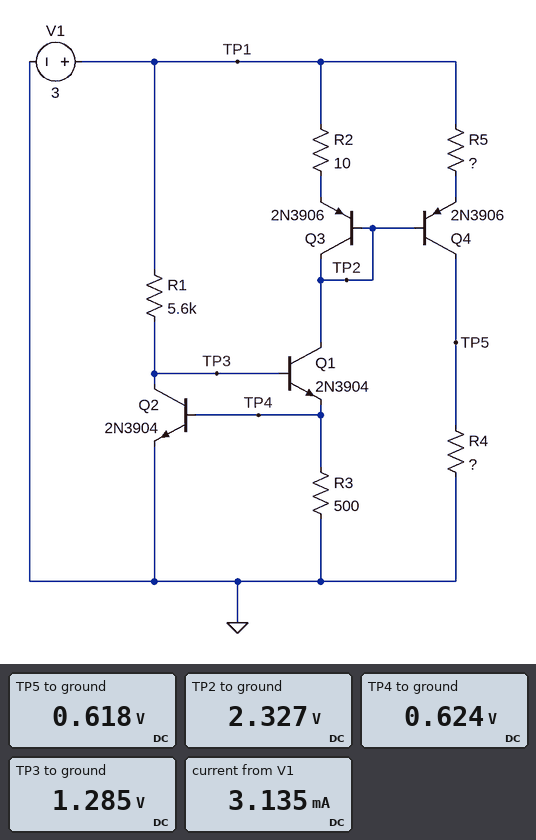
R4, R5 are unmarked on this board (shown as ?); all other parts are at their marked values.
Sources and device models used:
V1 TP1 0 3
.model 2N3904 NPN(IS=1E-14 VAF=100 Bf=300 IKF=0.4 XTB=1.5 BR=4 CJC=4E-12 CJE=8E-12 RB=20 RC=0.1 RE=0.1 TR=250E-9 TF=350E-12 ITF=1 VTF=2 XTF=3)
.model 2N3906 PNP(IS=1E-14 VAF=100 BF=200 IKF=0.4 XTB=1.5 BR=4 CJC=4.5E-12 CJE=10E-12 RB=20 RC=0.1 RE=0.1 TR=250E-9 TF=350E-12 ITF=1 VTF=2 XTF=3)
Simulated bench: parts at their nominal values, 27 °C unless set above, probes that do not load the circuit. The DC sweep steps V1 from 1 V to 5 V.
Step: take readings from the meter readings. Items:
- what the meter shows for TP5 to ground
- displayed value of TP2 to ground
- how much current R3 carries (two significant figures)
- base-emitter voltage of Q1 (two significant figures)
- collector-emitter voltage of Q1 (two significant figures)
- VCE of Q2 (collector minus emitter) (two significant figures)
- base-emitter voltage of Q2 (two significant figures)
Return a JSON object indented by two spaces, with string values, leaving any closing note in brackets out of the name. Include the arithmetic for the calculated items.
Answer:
{
  "what the meter shows for TP5 to ground": "0.618 V",
  "displayed value of TP2 to ground": "2.327 V",
  "how much current R3 carries": "(624 mV) / 500 Ω = 1.2 mA",
  "base-emitter voltage of Q1": "1.285 V - 624 mV = 660 mV",
  "collector-emitter voltage of Q1": "2.327 V - 624 mV = 1.7 V",
  "VCE of Q2 (collector minus emitter)": "1.285 V = 1.3 V",
  "base-emitter voltage of Q2": "624 mV = 620 mV"
}
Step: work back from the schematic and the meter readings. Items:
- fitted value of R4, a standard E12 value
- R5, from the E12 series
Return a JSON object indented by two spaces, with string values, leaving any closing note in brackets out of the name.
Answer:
{
  "fitted value of R4, a standard E12 value": "390 Ω",
  "R5, from the E12 series": "3.9 Ω"
}
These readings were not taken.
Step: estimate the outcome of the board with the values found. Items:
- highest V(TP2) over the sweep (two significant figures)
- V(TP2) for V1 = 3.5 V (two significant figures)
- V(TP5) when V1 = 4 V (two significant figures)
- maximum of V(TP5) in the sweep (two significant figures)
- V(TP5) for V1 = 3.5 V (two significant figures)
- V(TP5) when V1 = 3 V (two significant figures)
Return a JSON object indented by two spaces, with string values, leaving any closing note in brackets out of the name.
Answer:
{
  "highest V(TP2) over the sweep": "4.3 V",
  "V(TP2) for V1 = 3.5 V": "2.8 V",
  "V(TP5) when V1 = 4 V": "640 mV",
  "maximum of V(TP5) in the sweep": "650 mV",
  "V(TP5) for V1 = 3.5 V": "630 mV",
  "V(TP5) when V1 = 3 V": "620 mV"
}
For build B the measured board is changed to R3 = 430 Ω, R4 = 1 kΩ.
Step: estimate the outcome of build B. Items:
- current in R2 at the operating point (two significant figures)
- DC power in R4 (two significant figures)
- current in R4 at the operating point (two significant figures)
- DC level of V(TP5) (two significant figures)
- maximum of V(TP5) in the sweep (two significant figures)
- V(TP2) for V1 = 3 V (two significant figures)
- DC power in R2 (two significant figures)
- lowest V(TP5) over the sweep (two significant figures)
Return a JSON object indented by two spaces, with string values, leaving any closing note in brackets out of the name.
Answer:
{
  "current in R2 at the operating point": "1.4 mA",
  "DC power in R4": "3.5 mW",
  "current in R4 at the operating point": "1.9 mA",
  "DC level of V(TP5)": "1.9 V",
  "maximum of V(TP5) in the sweep": "2.0 V",
  "V(TP2) for V1 = 3 V": "2.3 V",
  "DC power in R2": "21 µW",
  "lowest V(TP5) over the sweep": "720 mV"
}
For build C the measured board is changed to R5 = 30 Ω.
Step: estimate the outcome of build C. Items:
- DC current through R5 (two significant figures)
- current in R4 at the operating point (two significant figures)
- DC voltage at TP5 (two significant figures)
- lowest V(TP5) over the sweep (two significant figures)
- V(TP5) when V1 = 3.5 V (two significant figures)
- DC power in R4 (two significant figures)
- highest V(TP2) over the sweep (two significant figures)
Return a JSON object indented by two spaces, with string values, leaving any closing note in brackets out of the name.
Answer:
{
  "DC current through R5": "810 µA",
  "current in R4 at the operating point": "800 µA",
  "DC voltage at TP5": "310 mV",
  "lowest V(TP5) over the sweep": "160 mV",
  "V(TP5) when V1 = 3.5 V": "320 mV",
  "DC power in R4": "250 µW",
  "highest V(TP2) over the sweep": "4.3 V"
}
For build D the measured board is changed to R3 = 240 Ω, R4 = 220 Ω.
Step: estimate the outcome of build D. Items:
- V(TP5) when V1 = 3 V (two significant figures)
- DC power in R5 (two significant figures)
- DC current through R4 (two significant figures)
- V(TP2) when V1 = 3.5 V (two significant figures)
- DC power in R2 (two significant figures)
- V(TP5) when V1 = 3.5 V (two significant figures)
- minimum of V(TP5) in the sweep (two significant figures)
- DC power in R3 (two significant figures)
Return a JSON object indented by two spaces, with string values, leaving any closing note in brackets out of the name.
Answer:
{
  "V(TP5) when V1 = 3 V": "850 mV",
  "DC power in R5": "59 µW",
  "DC current through R4": "3.9 mA",
  "V(TP2) when V1 = 3.5 V": "2.8 V",
  "DC power in R2": "66 µW",
  "V(TP5) when V1 = 3.5 V": "860 mV",
  "minimum of V(TP5) in the sweep": "280 mV",
  "DC power in R3": "1.6 mW"
}
